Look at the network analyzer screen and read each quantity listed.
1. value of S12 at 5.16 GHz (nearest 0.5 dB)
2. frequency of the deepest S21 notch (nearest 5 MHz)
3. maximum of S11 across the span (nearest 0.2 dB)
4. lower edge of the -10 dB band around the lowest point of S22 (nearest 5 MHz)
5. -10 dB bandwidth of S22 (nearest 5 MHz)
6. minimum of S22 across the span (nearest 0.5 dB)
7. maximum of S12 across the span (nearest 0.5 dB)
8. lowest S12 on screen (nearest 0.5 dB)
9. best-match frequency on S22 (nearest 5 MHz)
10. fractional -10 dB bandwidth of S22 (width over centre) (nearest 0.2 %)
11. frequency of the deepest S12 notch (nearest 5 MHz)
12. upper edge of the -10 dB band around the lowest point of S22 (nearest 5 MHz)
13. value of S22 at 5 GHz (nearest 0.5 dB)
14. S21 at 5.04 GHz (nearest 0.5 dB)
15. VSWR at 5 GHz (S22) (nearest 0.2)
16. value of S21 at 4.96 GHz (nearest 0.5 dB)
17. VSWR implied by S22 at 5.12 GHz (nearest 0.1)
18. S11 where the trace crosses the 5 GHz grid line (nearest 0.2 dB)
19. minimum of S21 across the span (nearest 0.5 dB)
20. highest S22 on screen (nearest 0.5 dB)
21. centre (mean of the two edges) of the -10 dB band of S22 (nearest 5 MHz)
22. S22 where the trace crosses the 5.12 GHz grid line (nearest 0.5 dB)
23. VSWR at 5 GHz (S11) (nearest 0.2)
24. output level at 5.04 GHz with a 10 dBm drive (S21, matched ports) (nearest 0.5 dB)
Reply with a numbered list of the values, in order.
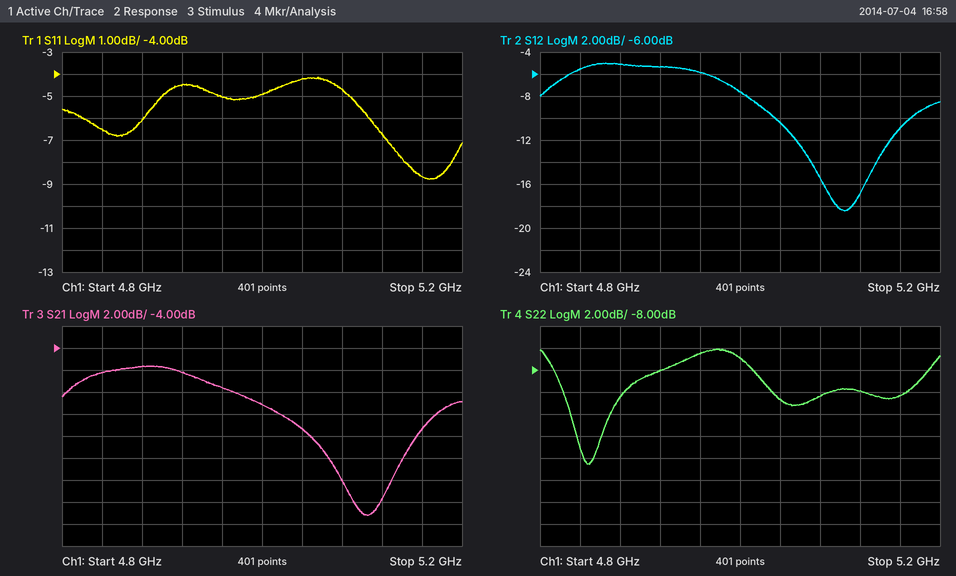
1. -11.0 dB
2. 5.105 GHz
3. -4.2 dB
4. 4.825 GHz
5. 60 MHz
6. -16.5 dB
7. -5.0 dB
8. -18.5 dB
9. 4.845 GHz
10. 1.2 %
11. 5.105 GHz
12. 4.885 GHz
13. -7.0 dB
14. -11.5 dB
15. 2.6
16. -7.5 dB
17. 1.9
18. -5.0 dB
19. -19.0 dB
20. -6.0 dB
21. 4.855 GHz
22. -10.0 dB
23. 3.6
24. -1.5 dBm
